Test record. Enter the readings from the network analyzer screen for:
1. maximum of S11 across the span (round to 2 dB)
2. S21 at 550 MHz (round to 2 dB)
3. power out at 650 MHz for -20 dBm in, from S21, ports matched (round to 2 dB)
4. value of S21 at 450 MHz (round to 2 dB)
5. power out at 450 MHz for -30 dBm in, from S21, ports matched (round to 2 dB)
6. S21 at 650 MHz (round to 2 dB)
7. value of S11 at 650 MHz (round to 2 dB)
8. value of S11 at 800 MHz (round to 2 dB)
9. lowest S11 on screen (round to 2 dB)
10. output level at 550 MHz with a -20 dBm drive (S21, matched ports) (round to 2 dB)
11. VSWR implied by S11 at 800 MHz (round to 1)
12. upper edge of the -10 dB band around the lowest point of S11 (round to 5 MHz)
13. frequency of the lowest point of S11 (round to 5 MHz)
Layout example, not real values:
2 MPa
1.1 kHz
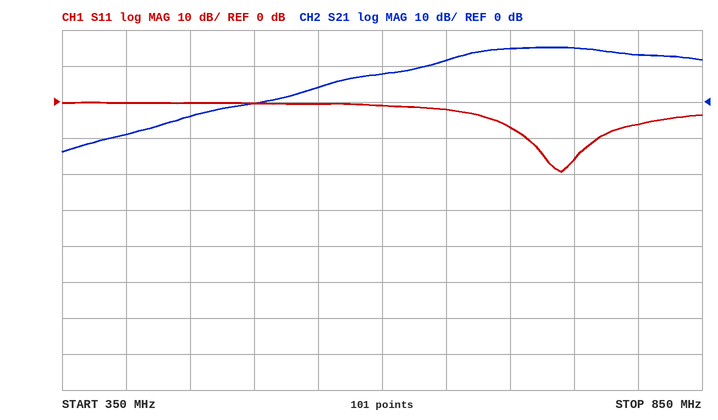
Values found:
0 dB
4 dB
-8 dBm
-4 dB
-34 dBm
12 dB
-2 dB
-6 dB
-20 dB
-16 dBm
3
770 MHz
740 MHz
